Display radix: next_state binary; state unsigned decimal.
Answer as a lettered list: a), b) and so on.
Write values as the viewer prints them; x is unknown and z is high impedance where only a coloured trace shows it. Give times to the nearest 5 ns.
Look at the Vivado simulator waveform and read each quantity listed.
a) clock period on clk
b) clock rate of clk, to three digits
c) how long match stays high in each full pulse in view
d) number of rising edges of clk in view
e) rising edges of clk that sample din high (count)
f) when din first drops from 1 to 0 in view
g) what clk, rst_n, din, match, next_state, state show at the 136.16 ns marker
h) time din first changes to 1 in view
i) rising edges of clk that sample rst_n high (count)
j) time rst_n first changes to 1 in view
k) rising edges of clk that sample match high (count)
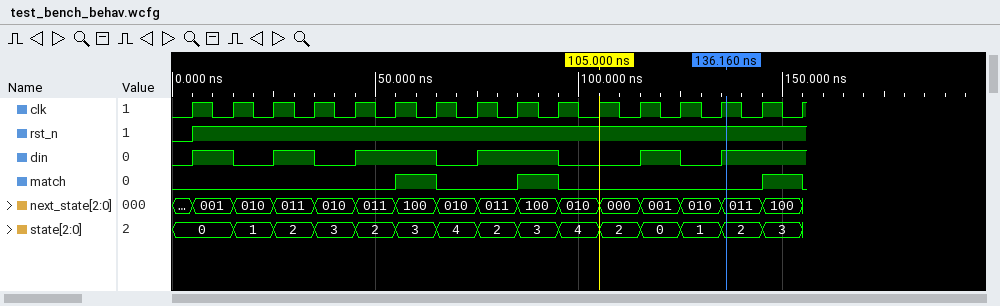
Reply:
a) 10 ns
b) 100 MHz
c) 10 ns, 10 ns, 10 ns
d) 16
e) 9
f) 15 ns
g) clk=1, rst_n=1, din=1, match=0, next_state=011, state=2
h) 5 ns
i) 15
j) 5 ns
k) 3
